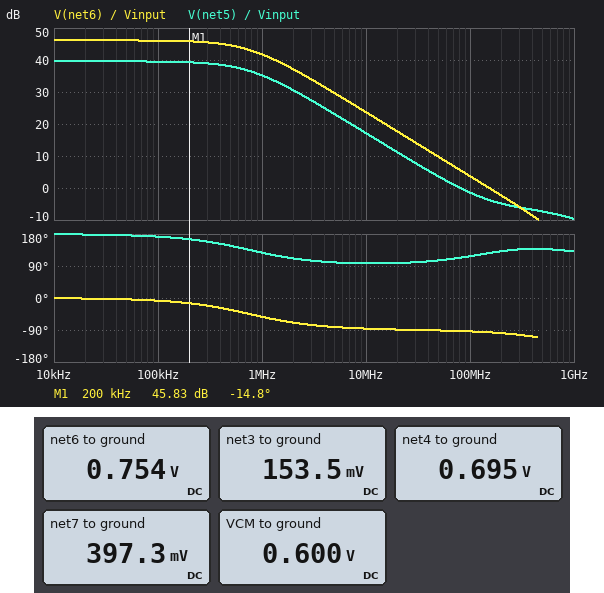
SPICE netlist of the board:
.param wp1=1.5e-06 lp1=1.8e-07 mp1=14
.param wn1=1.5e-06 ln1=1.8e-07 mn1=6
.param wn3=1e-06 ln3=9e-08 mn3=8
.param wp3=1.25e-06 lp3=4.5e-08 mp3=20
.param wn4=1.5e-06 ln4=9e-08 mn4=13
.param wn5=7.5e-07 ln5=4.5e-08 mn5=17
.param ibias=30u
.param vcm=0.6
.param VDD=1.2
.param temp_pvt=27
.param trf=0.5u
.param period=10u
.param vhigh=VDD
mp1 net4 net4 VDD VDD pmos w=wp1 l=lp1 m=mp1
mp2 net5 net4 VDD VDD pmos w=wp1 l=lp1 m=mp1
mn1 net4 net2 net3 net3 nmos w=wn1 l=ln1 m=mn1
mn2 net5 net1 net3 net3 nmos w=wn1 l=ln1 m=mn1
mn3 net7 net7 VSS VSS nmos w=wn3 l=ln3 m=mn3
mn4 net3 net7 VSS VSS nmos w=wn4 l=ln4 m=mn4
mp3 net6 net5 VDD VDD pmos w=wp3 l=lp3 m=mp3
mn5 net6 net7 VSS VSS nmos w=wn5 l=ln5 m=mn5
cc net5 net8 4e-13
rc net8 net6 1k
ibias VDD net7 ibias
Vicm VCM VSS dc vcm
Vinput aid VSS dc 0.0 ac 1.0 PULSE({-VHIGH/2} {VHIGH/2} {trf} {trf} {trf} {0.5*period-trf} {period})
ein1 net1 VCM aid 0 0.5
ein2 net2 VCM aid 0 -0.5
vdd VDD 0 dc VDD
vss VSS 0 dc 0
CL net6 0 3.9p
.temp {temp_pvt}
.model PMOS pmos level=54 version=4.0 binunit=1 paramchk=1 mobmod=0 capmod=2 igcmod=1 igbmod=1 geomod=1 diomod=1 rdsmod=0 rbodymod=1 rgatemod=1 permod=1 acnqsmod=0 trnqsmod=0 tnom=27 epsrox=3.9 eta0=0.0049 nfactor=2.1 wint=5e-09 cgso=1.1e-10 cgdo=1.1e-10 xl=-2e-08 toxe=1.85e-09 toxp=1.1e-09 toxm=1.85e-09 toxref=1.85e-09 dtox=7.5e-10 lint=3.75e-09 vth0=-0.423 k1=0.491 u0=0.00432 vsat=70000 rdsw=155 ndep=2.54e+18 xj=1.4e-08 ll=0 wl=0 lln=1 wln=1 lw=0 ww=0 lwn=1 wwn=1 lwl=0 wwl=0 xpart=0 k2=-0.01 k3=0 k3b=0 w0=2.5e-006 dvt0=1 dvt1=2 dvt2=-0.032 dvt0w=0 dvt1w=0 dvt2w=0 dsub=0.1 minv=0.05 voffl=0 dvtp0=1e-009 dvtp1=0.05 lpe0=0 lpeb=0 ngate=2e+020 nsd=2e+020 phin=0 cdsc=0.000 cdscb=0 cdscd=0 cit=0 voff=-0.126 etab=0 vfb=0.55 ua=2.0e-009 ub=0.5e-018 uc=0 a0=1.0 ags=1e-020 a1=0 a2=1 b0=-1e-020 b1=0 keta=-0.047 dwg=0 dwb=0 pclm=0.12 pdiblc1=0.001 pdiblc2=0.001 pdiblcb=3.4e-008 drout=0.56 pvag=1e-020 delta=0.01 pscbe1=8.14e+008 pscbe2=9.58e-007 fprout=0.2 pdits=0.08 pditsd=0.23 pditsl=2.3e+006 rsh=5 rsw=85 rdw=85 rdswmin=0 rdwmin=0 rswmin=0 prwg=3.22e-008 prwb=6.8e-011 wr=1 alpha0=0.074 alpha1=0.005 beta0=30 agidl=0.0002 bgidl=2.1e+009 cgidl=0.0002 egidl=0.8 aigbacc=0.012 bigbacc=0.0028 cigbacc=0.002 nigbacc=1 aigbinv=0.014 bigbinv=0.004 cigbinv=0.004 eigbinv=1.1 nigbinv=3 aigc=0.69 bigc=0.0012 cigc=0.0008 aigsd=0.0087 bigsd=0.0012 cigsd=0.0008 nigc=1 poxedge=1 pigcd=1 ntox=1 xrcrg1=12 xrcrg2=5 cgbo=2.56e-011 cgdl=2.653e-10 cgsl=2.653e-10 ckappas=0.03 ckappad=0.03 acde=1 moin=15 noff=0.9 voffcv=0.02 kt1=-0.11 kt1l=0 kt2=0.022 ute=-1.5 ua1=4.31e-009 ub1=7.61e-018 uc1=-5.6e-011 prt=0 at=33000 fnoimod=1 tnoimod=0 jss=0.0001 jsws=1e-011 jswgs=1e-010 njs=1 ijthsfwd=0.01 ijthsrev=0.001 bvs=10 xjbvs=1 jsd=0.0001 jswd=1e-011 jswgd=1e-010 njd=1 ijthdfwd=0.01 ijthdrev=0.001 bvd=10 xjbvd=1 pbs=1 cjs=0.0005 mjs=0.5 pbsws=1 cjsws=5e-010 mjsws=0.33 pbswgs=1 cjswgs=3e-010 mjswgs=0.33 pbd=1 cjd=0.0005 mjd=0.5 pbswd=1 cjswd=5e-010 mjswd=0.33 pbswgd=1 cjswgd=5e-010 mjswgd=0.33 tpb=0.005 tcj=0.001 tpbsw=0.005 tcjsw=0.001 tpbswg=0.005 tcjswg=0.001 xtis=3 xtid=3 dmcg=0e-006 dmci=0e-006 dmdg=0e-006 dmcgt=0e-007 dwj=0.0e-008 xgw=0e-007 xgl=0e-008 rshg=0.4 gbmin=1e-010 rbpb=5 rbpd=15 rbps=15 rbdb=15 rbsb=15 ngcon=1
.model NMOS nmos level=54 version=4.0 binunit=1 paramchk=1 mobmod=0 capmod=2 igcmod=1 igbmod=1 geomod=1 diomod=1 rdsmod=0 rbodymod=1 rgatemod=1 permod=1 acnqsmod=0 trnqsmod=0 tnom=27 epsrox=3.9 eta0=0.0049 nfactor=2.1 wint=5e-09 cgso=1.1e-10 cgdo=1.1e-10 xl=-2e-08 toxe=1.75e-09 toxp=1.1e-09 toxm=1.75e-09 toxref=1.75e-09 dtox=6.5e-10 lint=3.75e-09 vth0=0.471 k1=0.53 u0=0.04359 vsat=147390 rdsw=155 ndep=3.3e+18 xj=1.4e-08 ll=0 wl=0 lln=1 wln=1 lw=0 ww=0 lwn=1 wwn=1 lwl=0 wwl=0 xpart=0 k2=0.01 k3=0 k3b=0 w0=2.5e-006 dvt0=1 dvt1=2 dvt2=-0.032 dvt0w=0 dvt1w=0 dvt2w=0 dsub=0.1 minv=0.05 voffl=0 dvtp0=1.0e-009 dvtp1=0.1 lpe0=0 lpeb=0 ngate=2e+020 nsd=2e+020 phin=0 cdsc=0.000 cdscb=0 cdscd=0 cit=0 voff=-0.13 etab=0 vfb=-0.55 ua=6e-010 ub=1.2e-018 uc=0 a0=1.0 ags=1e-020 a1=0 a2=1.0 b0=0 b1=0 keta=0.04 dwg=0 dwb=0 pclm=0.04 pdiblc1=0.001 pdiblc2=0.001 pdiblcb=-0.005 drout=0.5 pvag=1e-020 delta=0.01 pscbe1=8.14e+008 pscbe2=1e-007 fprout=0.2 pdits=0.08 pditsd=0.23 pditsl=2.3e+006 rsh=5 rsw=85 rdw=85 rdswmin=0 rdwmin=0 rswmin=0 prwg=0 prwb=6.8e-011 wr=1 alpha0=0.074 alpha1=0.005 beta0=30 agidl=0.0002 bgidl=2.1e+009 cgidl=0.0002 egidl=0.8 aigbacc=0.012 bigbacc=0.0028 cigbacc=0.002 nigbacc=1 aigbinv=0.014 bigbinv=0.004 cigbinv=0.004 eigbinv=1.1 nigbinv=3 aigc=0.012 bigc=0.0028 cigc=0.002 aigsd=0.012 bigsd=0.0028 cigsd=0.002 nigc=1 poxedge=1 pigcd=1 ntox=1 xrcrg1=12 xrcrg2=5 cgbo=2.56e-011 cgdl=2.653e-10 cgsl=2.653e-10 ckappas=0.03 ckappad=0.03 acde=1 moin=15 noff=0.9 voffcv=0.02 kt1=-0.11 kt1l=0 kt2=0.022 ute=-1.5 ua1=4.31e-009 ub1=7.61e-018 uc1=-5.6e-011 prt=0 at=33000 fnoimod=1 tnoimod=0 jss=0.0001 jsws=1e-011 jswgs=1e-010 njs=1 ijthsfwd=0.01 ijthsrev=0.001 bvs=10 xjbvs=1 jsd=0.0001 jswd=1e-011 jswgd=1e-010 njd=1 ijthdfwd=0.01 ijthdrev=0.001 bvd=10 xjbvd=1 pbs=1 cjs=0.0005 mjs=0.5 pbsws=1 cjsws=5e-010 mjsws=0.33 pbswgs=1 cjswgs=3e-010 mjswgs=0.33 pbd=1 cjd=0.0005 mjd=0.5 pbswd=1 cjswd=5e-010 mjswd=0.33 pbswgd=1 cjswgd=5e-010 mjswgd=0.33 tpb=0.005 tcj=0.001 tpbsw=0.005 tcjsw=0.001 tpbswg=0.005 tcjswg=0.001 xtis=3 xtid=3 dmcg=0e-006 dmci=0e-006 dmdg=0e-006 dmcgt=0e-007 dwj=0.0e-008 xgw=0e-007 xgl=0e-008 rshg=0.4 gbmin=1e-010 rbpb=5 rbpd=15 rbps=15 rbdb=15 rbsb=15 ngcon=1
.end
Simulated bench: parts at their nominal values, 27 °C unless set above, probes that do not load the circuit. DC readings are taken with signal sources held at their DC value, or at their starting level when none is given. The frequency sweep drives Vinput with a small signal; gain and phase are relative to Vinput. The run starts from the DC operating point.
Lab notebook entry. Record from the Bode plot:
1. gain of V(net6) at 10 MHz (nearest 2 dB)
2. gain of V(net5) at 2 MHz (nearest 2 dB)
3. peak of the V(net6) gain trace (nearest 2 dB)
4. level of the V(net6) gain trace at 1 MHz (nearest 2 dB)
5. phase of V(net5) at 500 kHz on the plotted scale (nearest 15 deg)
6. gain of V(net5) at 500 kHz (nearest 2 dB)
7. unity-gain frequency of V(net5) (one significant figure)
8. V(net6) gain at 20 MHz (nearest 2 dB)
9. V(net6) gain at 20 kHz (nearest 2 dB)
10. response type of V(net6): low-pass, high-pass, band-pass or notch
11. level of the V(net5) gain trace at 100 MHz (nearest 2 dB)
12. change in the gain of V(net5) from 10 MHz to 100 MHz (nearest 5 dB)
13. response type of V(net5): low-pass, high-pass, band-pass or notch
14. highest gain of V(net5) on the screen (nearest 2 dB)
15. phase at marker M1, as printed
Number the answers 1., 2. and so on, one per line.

1. 24 dB
2. 30 dB
3. 46 dB
4. 42 dB
5. 150 deg
6. 38 dB
7. 80 MHz
8. 18 dB
9. 46 dB
10. low-pass
11. -2 dB
12. -20 dB
13. low-pass
14. 40 dB
15. -14.8 deg
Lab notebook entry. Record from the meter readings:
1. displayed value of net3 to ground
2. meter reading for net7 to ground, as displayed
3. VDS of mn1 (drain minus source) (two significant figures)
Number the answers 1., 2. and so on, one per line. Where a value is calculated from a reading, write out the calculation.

1. 153.5 mV
2. 397.3 mV
3. 695 mV - 153.5 mV = 540 mV
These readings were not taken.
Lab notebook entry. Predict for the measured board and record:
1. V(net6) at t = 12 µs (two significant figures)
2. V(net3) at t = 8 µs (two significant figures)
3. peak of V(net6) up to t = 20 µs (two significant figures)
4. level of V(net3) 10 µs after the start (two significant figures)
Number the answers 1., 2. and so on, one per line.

1. 1.1 V
2. 410 mV
3. 1.1 V
4. 410 mV
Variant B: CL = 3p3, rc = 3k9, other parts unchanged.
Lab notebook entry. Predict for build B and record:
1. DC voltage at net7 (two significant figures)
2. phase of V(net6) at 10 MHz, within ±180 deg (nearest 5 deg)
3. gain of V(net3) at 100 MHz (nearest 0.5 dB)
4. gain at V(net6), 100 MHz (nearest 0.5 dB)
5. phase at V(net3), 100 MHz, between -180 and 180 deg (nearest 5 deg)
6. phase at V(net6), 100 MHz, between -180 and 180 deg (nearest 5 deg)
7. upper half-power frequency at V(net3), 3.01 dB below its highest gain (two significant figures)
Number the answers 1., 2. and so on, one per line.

1. 400 mV
2. -80 deg
3. -41.0 dB
4. 6.5 dB
5. -170 deg
6. -65 deg
7. 750 kHz
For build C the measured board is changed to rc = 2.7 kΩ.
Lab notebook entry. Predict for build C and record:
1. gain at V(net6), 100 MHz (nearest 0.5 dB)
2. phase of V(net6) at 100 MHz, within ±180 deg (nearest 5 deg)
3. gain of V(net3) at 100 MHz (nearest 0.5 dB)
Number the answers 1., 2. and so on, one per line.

1. 5.0 dB
2. -75 deg
3. -42.0 dB
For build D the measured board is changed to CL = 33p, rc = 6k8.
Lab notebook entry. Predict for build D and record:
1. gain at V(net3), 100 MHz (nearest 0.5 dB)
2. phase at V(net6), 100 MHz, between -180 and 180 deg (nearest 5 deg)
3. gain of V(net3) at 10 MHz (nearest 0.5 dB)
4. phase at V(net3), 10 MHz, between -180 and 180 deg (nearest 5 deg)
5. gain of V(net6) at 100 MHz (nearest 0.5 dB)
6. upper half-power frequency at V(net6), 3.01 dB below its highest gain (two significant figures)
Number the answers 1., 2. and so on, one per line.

1. -36.5 dB
2. -105 deg
3. -33.0 dB
4. 130 deg
5. 4.0 dB
6. 740 kHz
